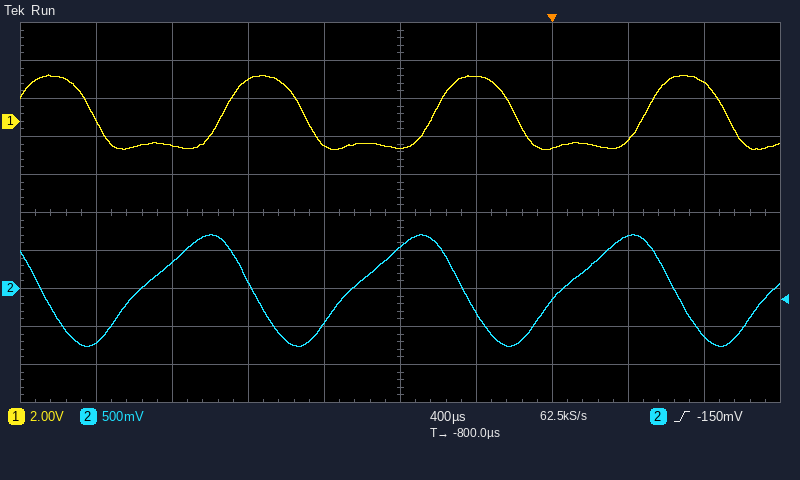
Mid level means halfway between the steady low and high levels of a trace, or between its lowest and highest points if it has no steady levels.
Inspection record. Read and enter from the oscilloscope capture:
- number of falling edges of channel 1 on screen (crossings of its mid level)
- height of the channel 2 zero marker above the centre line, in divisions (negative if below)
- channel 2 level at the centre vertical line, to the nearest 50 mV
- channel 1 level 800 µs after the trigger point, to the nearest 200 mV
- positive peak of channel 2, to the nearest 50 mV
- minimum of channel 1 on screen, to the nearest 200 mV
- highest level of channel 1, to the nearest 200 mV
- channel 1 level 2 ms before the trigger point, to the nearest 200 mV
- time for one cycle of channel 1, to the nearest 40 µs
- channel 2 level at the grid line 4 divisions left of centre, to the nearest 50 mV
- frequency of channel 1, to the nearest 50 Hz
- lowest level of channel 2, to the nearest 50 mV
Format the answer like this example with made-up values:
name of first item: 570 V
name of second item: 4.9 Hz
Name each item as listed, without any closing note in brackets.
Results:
number of falling edges of channel 1 on screen: 4
height of the channel 2 zero marker above the centre line, in divisions: -2.0 div
channel 2 level at the centre vertical line, to the nearest 50 mV: 550 mV
channel 1 level 800 µs after the trigger point, to the nearest 200 mV: 2.0 V
positive peak of channel 2, to the nearest 50 mV: 700 mV
minimum of channel 1 on screen, to the nearest 200 mV: -1.4 V
highest level of channel 1, to the nearest 200 mV: 2.4 V
channel 1 level 2 ms before the trigger point, to the nearest 200 mV: -1.2 V
time for one cycle of channel 1, to the nearest 40 µs: 1.12 ms
channel 2 level at the grid line 4 divisions left of centre, to the nearest 50 mV: -700 mV
frequency of channel 1, to the nearest 50 Hz: 900 Hz
lowest level of channel 2, to the nearest 50 mV: -750 mV
